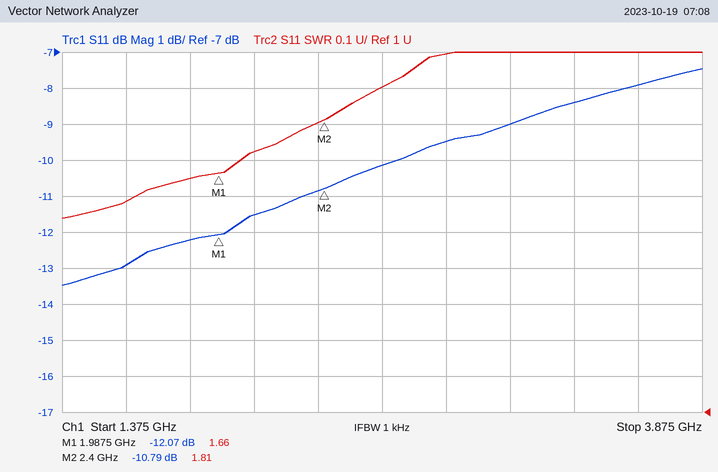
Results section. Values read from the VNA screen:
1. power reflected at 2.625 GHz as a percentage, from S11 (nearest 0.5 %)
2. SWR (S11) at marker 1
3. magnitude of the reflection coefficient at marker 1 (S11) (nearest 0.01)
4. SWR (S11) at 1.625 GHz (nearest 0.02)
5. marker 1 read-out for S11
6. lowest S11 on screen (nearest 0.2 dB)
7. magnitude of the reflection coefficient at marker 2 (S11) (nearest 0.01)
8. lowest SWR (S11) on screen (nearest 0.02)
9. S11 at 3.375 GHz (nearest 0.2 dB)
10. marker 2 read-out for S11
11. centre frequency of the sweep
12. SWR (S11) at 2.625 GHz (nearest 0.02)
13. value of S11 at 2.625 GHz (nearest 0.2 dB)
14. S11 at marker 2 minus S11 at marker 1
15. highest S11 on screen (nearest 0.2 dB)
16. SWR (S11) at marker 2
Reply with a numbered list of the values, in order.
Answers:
1. 9.5 %
2. 1.66
3. 0.25
4. 1.58
5. -12.07 dB
6. -13.4 dB
7. 0.29
8. 1.54
9. -8.4 dB
10. -10.79 dB
11. 2.625 GHz
12. 1.90
13. -10.2 dB
14. 1.28 dB
15. -7.4 dB
16. 1.81
